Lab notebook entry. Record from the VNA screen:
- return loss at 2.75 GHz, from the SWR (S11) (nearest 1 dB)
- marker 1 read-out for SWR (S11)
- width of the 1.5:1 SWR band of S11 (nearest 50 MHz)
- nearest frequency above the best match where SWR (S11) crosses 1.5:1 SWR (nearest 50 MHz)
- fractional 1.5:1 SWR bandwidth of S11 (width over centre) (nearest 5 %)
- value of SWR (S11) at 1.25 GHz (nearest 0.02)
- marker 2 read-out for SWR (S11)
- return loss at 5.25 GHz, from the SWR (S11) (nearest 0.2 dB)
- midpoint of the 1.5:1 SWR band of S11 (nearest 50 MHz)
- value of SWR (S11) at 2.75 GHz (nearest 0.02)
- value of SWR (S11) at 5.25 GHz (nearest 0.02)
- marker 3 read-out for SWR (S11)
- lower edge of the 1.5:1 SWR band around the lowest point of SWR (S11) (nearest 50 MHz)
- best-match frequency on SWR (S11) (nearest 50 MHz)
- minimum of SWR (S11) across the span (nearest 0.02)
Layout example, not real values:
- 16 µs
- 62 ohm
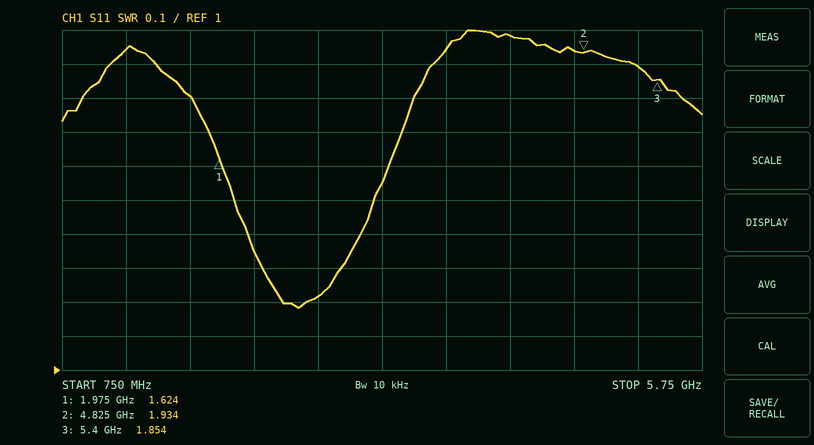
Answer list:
- 20 dB
- 1.624
- 1.10 GHz
- 3.20 GHz
- 40 %
- 1.94
- 1.934
- 10.2 dB
- 2.65 GHz
- 1.22
- 1.90
- 1.854
- 2.10 GHz
- 2.60 GHz
- 1.18
